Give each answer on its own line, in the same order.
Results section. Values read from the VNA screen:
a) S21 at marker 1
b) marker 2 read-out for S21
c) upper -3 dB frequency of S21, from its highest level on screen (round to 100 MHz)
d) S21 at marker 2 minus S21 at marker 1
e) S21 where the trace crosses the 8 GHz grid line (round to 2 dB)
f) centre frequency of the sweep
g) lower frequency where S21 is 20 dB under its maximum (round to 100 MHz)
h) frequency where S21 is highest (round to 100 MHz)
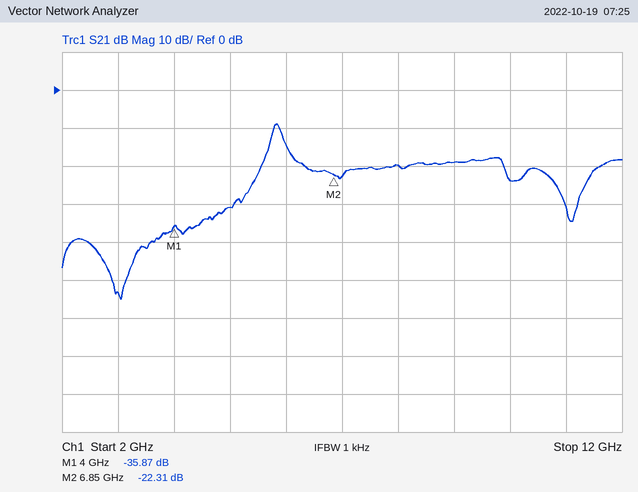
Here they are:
-35.87 dB
-22.31 dB
5.9 GHz
13.56 dB
-20 dB
7 GHz
5.2 GHz
5.8 GHz
